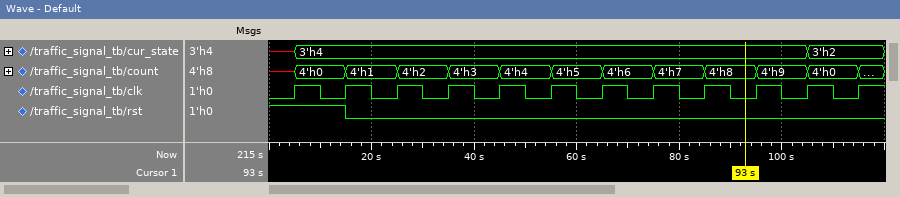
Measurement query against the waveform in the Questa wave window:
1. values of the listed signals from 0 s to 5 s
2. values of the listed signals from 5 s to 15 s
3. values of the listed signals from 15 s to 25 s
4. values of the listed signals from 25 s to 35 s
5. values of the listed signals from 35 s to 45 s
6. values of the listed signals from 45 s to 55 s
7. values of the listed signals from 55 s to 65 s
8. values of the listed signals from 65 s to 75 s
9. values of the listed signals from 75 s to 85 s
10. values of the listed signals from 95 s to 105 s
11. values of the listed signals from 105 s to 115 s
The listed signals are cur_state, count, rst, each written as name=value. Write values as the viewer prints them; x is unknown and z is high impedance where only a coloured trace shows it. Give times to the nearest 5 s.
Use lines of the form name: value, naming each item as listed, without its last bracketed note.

values of the listed signals from 0 s to 5 s: cur_state=x, count=x, rst=1
values of the listed signals from 5 s to 15 s: cur_state=3'h4, count=4'h0, rst=1
values of the listed signals from 15 s to 25 s: cur_state=3'h4, count=4'h1, rst=0
values of the listed signals from 25 s to 35 s: cur_state=3'h4, count=4'h2, rst=0
values of the listed signals from 35 s to 45 s: cur_state=3'h4, count=4'h3, rst=0
values of the listed signals from 45 s to 55 s: cur_state=3'h4, count=4'h4, rst=0
values of the listed signals from 55 s to 65 s: cur_state=3'h4, count=4'h5, rst=0
values of the listed signals from 65 s to 75 s: cur_state=3'h4, count=4'h6, rst=0
values of the listed signals from 75 s to 85 s: cur_state=3'h4, count=4'h7, rst=0
values of the listed signals from 95 s to 105 s: cur_state=3'h4, count=4'h9, rst=0
values of the listed signals from 105 s to 115 s: cur_state=3'h2, count=4'h0, rst=0
